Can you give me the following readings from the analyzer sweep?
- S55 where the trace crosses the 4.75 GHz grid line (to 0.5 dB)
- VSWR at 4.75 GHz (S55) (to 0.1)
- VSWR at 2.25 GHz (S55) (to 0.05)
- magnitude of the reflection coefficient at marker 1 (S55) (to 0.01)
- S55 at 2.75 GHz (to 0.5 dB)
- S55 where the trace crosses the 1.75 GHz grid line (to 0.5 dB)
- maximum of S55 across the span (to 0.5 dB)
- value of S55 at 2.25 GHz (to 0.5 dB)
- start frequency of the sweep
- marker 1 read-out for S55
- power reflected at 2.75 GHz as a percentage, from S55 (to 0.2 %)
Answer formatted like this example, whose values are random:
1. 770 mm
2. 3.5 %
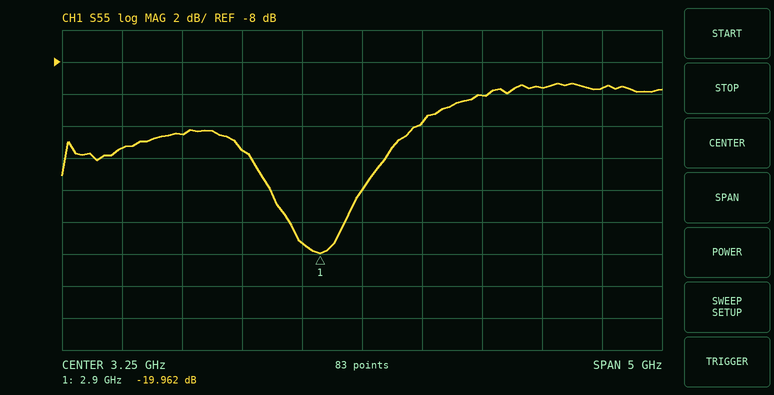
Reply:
1. -9.5 dB
2. 2.0
3. 1.55
4. 0.10
5. -19.5 dB
6. -12.5 dB
7. -9.5 dB
8. -13.5 dB
9. 750 MHz
10. -19.962 dB
11. 1.2 %
